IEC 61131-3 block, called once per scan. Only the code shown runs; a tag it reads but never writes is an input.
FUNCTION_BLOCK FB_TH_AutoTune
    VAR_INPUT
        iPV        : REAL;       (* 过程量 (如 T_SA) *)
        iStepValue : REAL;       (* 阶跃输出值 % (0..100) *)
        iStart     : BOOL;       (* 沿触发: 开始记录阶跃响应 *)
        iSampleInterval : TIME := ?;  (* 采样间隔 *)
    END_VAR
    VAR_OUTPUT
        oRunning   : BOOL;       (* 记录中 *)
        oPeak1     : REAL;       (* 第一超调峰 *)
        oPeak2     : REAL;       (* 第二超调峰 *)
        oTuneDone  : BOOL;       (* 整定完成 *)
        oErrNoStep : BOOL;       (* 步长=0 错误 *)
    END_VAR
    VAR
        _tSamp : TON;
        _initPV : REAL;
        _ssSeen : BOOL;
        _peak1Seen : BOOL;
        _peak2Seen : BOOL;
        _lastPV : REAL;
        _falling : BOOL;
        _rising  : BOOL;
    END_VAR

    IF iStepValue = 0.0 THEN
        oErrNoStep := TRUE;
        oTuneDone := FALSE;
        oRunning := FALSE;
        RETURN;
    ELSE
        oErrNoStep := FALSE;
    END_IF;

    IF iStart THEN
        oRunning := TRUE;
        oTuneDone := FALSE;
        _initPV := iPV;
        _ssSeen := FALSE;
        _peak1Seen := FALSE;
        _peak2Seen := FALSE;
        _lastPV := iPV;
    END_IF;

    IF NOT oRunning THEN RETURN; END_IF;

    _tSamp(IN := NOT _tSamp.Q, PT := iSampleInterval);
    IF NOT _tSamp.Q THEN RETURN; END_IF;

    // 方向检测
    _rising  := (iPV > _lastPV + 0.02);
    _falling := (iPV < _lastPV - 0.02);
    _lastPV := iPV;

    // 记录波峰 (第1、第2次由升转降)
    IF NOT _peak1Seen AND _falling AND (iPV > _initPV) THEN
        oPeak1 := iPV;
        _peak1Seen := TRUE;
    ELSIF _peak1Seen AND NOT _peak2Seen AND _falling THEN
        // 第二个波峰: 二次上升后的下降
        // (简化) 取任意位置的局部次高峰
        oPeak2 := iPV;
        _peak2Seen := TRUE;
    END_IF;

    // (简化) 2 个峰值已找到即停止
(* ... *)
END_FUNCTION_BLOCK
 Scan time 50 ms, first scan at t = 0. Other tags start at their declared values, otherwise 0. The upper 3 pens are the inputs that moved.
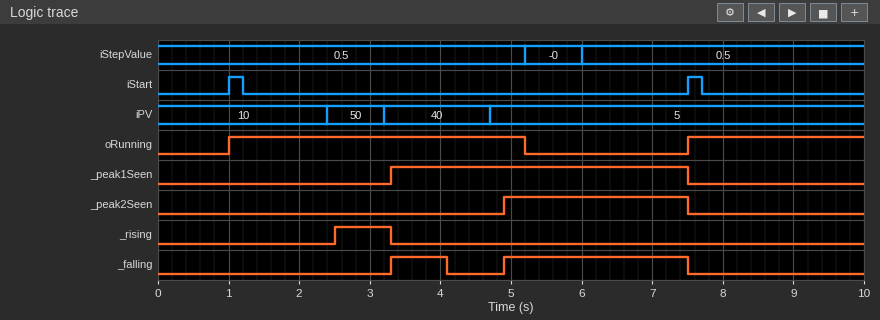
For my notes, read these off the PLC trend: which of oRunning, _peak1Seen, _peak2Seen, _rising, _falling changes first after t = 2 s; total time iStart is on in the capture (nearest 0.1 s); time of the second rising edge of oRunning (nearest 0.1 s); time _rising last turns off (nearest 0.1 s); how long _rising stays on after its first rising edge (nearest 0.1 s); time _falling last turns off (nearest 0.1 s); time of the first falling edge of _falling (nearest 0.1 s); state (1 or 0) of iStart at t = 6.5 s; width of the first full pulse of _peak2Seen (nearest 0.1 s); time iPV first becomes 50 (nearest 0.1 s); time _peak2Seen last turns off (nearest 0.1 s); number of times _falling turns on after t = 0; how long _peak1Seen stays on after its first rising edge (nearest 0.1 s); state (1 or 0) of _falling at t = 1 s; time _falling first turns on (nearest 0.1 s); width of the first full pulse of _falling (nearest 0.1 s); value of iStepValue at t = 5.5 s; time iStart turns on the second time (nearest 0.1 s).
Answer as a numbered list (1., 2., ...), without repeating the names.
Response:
1. _rising
2. 0.4 s
3. 7.5 s
4. 3.3 s
5. 0.8 s
6. 7.5 s
7. 4.1 s
8. 0
9. 2.6 s
10. 2.4 s
11. 7.5 s
12. 2
13. 4.2 s
14. 0
15. 3.3 s
16. 0.8 s
17. -0
18. 7.5 s
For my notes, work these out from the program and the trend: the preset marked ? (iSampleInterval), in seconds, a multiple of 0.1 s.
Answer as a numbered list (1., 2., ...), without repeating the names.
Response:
1. 0.7 s
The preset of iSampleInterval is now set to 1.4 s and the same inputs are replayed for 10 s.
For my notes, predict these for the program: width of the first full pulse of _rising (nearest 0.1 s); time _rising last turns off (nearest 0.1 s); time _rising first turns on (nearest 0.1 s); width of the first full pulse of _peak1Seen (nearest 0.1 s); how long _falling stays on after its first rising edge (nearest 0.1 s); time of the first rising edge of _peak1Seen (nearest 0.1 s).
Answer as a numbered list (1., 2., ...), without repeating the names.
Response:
1. 1.5 s
2. 3.9 s
3. 2.4 s
4. 3.6 s
5. 3.6 s
6. 3.9 s
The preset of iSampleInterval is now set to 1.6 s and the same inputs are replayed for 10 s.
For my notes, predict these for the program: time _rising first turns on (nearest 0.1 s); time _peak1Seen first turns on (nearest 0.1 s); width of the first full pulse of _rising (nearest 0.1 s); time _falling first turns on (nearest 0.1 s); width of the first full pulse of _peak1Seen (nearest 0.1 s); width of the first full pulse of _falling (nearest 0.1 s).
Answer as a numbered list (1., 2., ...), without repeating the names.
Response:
1. 2.6 s
2. 4.3 s
3. 1.7 s
4. 4.3 s
5. 3.2 s
6. 3.2 s
